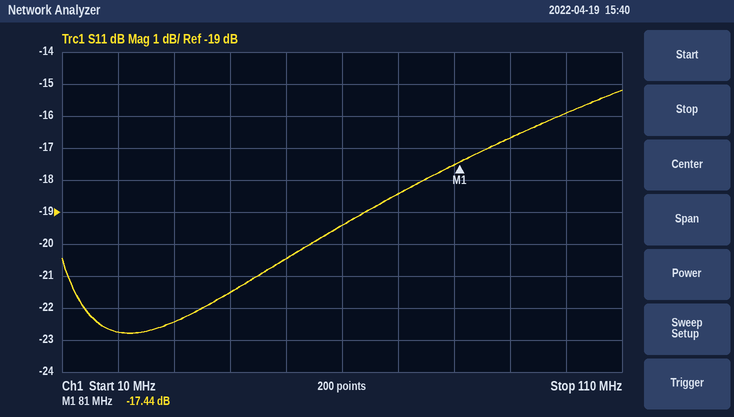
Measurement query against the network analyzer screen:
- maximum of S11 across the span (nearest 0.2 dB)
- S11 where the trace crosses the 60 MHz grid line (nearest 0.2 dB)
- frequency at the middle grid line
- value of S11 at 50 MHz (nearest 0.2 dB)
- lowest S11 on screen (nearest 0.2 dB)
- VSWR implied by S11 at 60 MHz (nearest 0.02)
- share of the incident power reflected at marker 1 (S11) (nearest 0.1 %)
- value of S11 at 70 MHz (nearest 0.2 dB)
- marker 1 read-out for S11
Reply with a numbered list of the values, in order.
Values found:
1. -15.2 dB
2. -19.4 dB
3. 60 MHz
4. -20.4 dB
5. -22.8 dB
6. 1.24
7. 1.8 %
8. -18.4 dB
9. -17.44 dB
